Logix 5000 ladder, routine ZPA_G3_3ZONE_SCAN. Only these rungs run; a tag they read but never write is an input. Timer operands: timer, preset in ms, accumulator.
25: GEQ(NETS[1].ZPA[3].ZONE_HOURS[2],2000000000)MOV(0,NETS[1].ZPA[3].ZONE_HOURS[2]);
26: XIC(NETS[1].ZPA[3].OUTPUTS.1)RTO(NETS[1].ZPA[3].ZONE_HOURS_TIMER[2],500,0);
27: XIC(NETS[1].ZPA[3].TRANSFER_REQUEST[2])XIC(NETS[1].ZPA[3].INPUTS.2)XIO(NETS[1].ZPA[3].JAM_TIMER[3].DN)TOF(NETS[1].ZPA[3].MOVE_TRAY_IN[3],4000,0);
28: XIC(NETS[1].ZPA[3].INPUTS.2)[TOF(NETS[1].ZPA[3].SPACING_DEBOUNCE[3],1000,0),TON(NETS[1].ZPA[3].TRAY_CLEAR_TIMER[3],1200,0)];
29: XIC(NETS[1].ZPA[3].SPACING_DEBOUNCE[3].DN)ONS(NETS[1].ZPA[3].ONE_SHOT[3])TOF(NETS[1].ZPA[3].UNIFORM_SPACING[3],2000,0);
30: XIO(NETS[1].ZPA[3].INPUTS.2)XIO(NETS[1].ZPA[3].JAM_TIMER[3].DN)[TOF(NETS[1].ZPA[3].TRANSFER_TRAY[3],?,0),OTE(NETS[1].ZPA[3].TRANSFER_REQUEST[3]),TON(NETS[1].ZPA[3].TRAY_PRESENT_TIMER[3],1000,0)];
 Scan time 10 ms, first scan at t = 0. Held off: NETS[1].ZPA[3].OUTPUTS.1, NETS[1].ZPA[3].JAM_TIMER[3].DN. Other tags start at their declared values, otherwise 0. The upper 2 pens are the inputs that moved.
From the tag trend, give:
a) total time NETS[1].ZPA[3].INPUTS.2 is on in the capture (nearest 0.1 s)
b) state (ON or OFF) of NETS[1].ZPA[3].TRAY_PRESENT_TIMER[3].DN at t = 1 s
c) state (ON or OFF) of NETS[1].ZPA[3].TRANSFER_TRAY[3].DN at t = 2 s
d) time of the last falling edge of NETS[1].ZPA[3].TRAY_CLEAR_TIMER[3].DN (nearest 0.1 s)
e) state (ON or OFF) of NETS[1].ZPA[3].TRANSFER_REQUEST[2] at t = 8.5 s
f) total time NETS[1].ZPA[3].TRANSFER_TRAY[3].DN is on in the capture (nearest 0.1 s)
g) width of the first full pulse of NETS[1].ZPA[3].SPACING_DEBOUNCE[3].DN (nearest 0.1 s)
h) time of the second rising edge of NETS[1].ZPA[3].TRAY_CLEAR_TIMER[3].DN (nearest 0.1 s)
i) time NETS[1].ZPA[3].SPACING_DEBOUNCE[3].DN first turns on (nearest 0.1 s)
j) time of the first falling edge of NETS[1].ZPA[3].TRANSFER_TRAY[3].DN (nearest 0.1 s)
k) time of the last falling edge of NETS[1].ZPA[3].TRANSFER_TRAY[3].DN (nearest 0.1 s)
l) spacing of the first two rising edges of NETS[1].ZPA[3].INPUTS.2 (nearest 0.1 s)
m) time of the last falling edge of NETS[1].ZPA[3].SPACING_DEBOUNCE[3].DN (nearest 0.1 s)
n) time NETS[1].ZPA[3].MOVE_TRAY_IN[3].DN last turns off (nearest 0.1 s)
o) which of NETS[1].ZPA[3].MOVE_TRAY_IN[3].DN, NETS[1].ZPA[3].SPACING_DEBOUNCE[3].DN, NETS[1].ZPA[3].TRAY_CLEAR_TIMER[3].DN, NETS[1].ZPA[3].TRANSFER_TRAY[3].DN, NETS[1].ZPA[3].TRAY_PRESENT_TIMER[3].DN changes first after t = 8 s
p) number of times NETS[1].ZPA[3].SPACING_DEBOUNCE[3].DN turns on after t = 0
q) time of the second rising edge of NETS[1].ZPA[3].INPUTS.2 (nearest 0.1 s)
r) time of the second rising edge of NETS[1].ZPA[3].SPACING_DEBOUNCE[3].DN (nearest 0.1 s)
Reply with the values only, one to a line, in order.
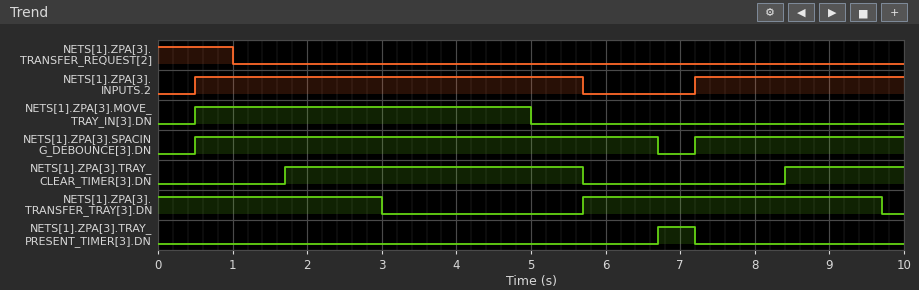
8.0 s
OFF
ON
5.7 s
OFF
7.0 s
6.2 s
8.4 s
0.5 s
3.0 s
9.7 s
6.7 s
6.7 s
5.0 s
NETS[1].ZPA[3].TRAY_CLEAR_TIMER[3].DN
2
7.2 s
7.2 s
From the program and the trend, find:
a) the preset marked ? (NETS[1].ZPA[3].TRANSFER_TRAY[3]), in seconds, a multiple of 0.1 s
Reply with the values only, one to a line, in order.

2.5 s
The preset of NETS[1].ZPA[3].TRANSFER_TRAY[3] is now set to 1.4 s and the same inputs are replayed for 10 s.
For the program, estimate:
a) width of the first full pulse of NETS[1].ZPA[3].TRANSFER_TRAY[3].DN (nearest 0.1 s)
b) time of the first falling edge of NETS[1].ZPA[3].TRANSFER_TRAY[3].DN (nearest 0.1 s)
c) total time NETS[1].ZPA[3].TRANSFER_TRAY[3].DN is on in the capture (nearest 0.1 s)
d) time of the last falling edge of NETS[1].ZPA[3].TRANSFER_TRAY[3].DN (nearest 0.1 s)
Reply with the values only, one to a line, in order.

2.9 s
1.9 s
4.8 s
8.6 s
